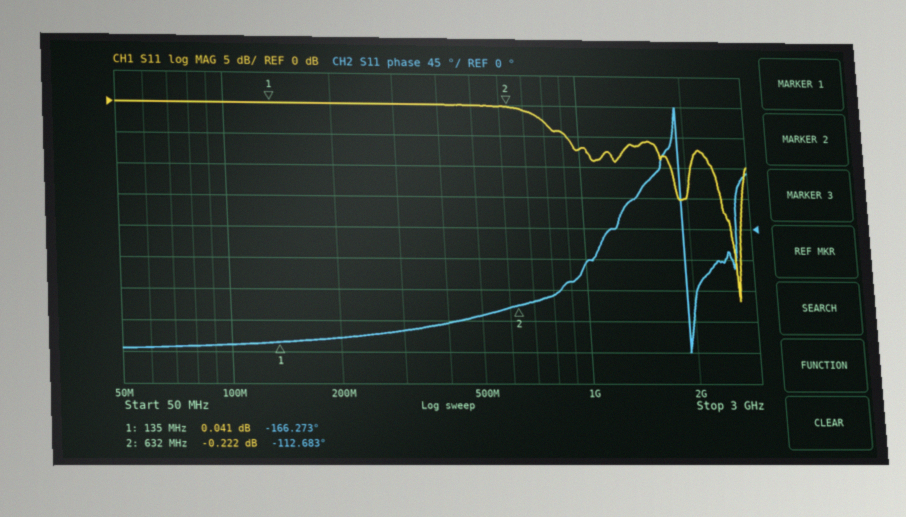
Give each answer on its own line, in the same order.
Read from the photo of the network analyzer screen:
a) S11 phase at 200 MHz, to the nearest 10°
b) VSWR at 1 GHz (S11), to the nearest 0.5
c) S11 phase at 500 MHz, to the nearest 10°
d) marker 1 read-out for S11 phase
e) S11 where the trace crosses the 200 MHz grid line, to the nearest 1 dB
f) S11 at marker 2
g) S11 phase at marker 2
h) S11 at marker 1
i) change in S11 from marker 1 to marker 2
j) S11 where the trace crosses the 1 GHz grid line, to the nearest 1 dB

-160°
2.5
-130°
-166.273°
0 dB
-0.222 dB
-112.683°
0.041 dB
-0.263 dB
-7 dB
